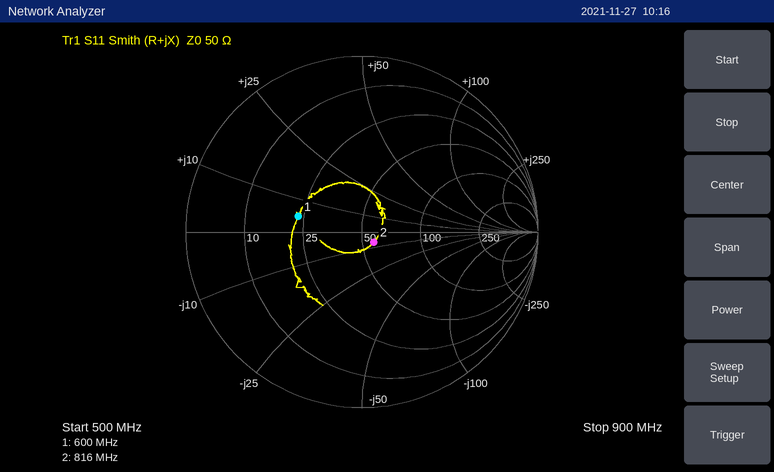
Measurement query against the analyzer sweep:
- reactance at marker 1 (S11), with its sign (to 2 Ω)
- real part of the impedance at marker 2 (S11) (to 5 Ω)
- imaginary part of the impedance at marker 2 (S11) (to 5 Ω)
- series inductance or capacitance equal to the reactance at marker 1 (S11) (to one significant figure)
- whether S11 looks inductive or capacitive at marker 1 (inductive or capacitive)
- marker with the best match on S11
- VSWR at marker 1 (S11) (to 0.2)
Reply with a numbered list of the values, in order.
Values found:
1. +4 Ω
2. 55 Ω
3. -5 Ω
4. 1 nH
5. inductive
6. marker 2
7. 2.2
